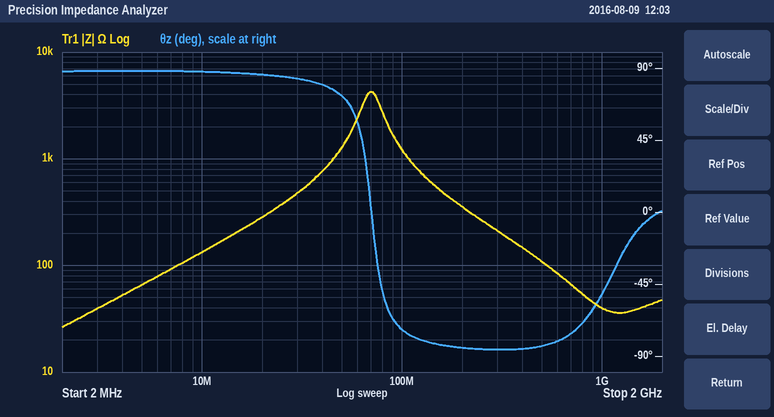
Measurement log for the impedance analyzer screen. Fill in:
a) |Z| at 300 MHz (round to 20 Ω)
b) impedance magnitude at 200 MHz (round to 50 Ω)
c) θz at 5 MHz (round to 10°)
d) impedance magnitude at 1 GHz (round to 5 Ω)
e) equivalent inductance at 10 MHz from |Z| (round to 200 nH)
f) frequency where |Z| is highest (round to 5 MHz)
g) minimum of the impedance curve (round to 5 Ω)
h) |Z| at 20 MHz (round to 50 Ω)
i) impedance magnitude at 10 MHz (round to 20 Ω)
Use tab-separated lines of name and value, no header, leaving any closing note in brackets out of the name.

|Z| at 300 MHz	220 Ω
impedance magnitude at 200 MHz	350 Ω
θz at 5 MHz	90°
impedance magnitude at 1 GHz	40 Ω
equivalent inductance at 10 MHz from |Z|	2.2 µH
frequency where |Z| is highest	70 MHz
minimum of the impedance curve	25 Ω
|Z| at 20 MHz	300 Ω
impedance magnitude at 10 MHz	140 Ω
